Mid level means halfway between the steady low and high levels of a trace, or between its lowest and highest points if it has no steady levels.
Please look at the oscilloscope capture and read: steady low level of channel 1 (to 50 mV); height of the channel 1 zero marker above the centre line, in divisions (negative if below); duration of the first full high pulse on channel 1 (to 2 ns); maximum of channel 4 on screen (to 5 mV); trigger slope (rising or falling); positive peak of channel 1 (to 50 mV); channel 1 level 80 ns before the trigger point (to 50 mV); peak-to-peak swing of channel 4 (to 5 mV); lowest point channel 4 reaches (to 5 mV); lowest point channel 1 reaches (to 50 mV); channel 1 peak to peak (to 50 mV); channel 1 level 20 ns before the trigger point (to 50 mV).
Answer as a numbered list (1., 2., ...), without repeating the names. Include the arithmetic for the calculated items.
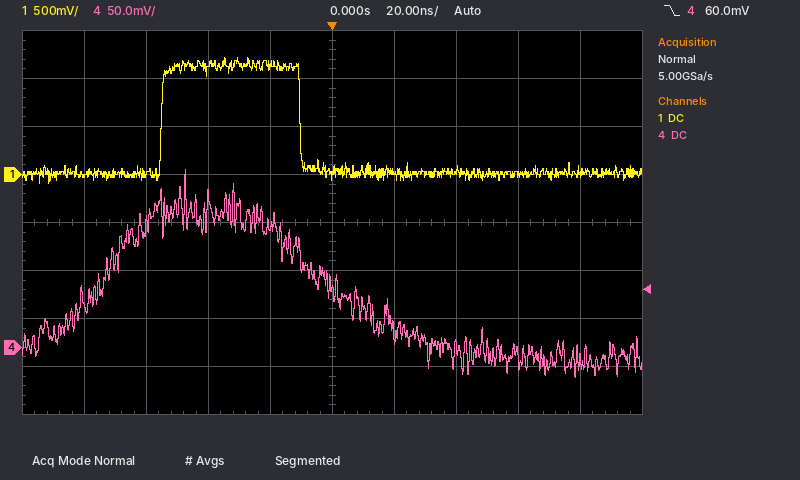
1. 0 mV
2. +1.0 div
3. 44 ns
4. 185 mV
5. falling
6. 1.20 V
7. 0 mV
8. 185 mV − (-30 mV) = 215 mV
9. -30 mV
10. -100 mV
11. 1.20 V − (-100 mV) = 1.30 V
12. 1.15 V
